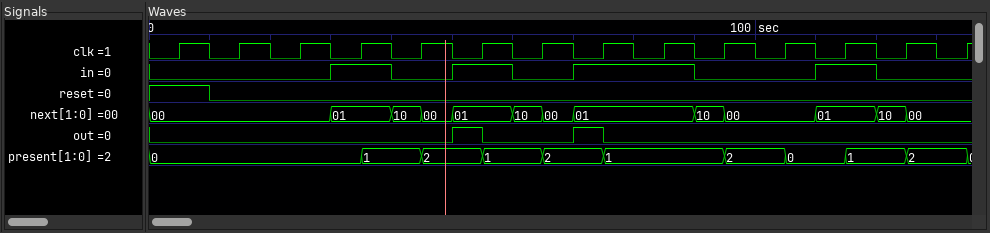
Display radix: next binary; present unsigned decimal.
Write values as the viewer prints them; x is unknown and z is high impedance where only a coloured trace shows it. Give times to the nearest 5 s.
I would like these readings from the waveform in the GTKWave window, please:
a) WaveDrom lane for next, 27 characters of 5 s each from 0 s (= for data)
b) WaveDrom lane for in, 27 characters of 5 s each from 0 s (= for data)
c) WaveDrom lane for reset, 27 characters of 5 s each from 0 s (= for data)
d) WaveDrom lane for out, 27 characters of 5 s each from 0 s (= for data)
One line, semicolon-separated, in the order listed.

{name: 'next', wave: '=.....=.===.===...==..=.==.', data: '00 01 10 00 01 10 00 01 10 00 01 10 00'}; {name: 'in', wave: '0.....1.0.1.0.1...0...1.0..'}; {name: 'reset', wave: '1.0........................'}; {name: 'out', wave: '0.........10..10...........'}
